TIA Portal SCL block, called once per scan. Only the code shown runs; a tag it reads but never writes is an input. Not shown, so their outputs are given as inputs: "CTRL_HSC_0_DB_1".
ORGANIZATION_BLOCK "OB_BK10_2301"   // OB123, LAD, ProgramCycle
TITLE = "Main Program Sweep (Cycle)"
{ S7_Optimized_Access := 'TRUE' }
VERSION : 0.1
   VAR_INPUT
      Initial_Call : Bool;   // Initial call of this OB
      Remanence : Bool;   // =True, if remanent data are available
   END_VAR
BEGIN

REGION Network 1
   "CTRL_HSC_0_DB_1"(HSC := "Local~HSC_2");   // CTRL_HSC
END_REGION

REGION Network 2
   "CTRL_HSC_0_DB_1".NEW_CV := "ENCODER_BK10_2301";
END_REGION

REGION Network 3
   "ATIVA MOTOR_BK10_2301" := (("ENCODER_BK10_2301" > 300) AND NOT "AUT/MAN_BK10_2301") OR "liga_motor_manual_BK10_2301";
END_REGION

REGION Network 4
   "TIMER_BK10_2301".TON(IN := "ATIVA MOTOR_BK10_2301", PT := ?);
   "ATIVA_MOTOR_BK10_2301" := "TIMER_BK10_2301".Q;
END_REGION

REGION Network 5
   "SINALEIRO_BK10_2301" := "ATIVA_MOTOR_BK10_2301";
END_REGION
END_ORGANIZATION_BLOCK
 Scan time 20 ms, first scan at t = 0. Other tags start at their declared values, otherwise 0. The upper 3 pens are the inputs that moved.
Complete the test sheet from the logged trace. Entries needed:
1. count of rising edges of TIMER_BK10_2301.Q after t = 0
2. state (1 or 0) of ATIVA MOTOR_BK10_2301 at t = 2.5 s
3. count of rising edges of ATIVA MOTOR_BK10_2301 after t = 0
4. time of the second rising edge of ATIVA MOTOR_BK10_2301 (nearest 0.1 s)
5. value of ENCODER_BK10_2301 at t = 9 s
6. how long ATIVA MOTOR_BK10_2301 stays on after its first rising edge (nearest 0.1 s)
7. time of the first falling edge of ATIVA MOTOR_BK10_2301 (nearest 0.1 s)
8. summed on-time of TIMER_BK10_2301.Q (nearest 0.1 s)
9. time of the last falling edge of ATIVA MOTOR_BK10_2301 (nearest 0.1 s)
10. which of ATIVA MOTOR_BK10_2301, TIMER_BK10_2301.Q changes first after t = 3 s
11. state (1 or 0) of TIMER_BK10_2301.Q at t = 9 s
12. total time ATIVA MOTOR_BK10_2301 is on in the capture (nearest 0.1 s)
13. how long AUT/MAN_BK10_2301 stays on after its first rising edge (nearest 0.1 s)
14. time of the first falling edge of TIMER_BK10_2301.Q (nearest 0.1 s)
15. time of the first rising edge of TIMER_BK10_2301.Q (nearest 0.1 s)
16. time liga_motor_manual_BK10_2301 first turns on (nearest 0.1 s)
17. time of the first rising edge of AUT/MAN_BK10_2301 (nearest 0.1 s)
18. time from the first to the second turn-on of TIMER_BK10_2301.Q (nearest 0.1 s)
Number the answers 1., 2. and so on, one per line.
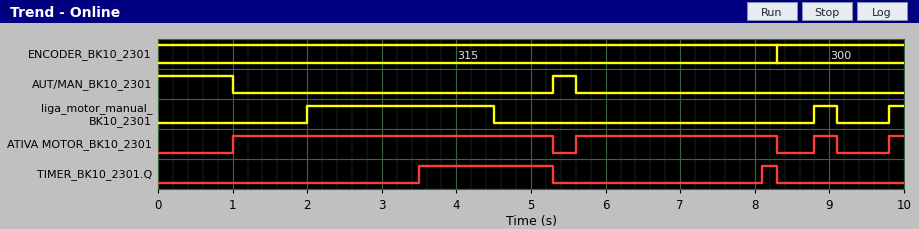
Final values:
1. 2
2. 1
3. 4
4. 5.6 s
5. 300
6. 4.3 s
7. 5.3 s
8. 2.0 s
9. 9.1 s
10. TIMER_BK10_2301.Q
11. 0
12. 7.5 s
13. 0.3 s
14. 5.3 s
15. 3.5 s
16. 2.0 s
17. 5.3 s
18. 4.6 s
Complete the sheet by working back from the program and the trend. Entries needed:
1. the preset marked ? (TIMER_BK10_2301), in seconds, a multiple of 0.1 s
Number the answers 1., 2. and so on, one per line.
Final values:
1. 2.5 s
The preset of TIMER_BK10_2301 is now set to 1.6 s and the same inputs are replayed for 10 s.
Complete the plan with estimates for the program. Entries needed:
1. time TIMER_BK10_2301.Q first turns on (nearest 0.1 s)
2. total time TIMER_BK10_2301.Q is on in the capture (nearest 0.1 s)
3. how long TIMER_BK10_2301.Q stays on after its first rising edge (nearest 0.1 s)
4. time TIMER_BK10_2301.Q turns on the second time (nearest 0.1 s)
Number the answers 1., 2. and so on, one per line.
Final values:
1. 2.6 s
2. 3.8 s
3. 2.7 s
4. 7.2 s
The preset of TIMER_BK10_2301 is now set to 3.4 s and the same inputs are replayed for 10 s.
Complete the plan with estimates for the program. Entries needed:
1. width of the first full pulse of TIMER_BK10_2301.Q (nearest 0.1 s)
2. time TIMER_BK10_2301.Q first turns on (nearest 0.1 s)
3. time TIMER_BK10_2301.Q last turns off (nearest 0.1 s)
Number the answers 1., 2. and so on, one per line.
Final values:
1. 0.9 s
2. 4.4 s
3. 5.3 s
